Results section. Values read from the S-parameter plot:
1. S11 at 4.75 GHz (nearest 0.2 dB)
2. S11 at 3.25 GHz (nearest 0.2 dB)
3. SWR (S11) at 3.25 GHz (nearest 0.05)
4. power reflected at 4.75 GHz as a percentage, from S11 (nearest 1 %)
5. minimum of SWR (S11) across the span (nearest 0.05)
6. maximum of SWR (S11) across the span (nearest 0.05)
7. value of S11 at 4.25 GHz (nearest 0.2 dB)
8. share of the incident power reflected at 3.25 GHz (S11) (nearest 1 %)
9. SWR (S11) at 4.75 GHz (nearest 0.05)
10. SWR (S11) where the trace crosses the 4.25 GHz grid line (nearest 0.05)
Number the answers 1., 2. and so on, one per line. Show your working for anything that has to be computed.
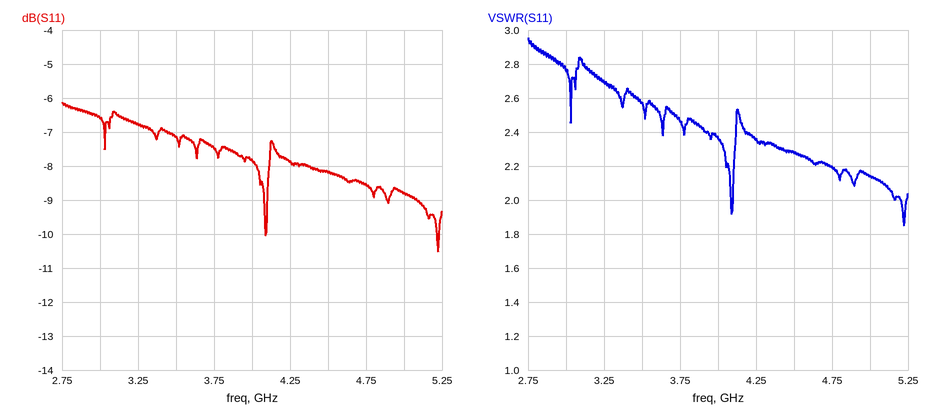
1. -8.6 dB
2. -6.8 dB
3. 2.70
4. 10^(-8.6/10) ≈ 14 %
5. 1.85
6. 2.95
7. -7.8 dB
8. 10^(-6.8/10) ≈ 21 %
9. 2.20
10. 2.35
